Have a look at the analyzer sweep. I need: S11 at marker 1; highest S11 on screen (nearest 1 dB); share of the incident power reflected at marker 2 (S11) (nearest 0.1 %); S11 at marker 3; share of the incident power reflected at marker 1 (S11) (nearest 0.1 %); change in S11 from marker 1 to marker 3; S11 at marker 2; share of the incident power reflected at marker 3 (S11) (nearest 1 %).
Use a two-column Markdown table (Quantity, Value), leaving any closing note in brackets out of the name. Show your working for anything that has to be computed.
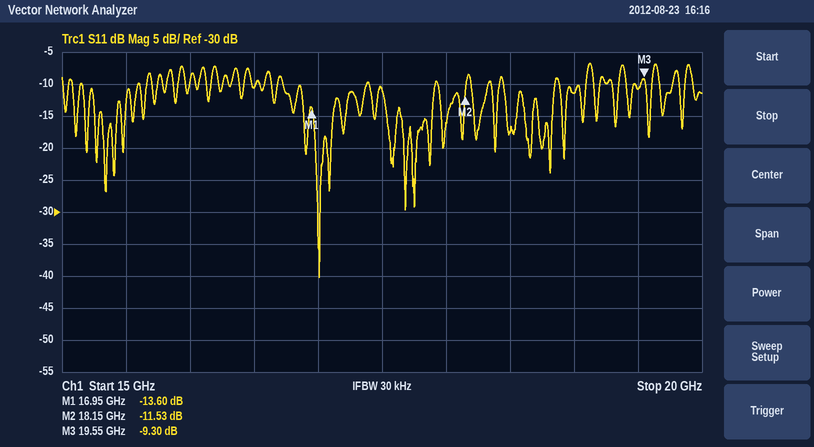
| Quantity | Value |
|---|---|
| S11 at marker 1 | -13.60 dB |
| highest S11 on screen | -7 dB |
| share of the incident power reflected at marker 2 (S11) | 10^(-11.53/10) ≈ 7.0 % |
| S11 at marker 3 | -9.30 dB |
| share of the incident power reflected at marker 1 (S11) | 10^(-13.6/10) ≈ 4.4 % |
| change in S11 from marker 1 to marker 3 | -9.3 − (-13.6) = 4.30 dB |
| S11 at marker 2 | -11.53 dB |
| share of the incident power reflected at marker 3 (S11) | 10^(-9.3/10) ≈ 12 % |
